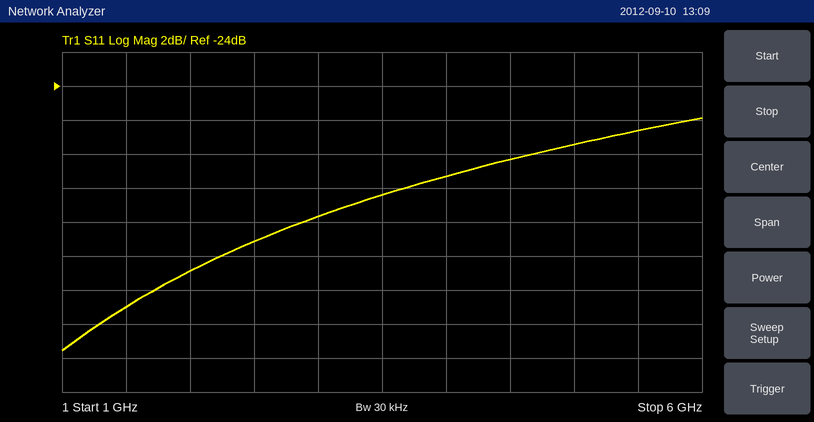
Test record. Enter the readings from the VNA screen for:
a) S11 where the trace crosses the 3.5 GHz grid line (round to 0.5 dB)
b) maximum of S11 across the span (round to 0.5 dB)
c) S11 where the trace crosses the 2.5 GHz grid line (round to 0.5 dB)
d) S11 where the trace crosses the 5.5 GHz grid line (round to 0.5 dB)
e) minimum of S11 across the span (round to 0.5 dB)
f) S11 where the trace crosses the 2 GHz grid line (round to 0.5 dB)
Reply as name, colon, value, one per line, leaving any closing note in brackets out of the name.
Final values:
S11 where the trace crosses the 3.5 GHz grid line: -30.5 dB
maximum of S11 across the span: -26.0 dB
S11 where the trace crosses the 2.5 GHz grid line: -33.0 dB
S11 where the trace crosses the 5.5 GHz grid line: -26.5 dB
minimum of S11 across the span: -39.5 dB
S11 where the trace crosses the 2 GHz grid line: -35.0 dB
